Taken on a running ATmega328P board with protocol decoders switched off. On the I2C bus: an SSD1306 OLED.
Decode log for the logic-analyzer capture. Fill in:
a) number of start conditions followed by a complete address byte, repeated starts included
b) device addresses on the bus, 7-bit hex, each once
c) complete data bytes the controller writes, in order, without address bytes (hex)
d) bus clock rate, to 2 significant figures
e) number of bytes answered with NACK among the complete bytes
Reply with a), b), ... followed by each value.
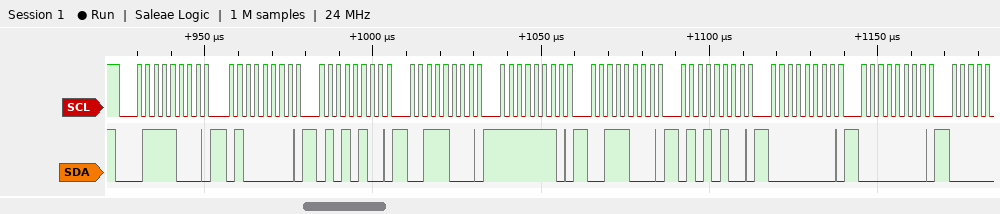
a) 1
b) 0x3C
c) 40 54 38 FE 38 54 00 00
d) 400 kHz
e) 0
